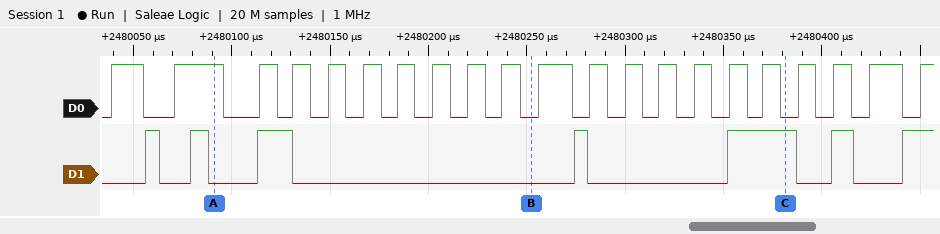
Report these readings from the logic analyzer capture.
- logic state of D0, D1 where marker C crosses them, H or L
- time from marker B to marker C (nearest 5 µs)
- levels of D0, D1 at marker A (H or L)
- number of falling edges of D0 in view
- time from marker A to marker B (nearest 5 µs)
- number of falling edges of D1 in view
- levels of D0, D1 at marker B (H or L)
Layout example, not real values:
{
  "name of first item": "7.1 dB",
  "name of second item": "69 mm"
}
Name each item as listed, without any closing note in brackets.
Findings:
{
  "logic state of D0, D1 where marker C crosses them, H or L": "D0=L, D1=H",
  "time from marker B to marker C": "130 µs",
  "levels of D0, D1 at marker A": "D0=H, D1=L",
  "number of falling edges of D0 in view": "20",
  "time from marker A to marker B": "160 µs",
  "number of falling edges of D1 in view": "6",
  "levels of D0, D1 at marker B": "D0=L, D1=L"
}
